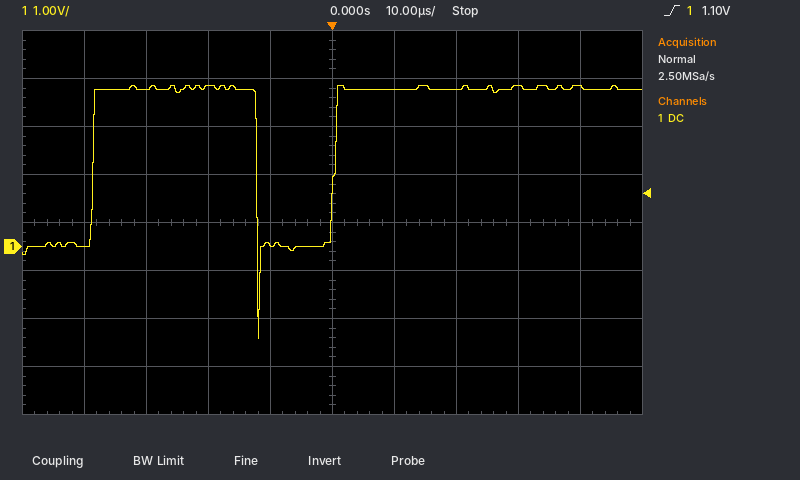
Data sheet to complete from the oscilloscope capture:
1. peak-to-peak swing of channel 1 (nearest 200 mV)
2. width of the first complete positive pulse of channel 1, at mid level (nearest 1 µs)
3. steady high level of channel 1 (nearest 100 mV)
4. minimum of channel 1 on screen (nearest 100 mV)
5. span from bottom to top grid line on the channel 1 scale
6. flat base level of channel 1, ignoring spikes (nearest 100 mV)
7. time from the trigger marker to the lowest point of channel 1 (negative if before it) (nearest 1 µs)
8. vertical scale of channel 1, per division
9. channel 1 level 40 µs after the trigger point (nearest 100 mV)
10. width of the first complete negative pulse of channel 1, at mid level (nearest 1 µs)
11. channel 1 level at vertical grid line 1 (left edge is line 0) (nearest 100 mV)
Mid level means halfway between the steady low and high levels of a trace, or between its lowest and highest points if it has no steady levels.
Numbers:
5.2 V
26 µs
3.3 V
-1.9 V
8 V
0.0 V
-12 µs
1 V
3.3 V
13 µs
0.0 V
